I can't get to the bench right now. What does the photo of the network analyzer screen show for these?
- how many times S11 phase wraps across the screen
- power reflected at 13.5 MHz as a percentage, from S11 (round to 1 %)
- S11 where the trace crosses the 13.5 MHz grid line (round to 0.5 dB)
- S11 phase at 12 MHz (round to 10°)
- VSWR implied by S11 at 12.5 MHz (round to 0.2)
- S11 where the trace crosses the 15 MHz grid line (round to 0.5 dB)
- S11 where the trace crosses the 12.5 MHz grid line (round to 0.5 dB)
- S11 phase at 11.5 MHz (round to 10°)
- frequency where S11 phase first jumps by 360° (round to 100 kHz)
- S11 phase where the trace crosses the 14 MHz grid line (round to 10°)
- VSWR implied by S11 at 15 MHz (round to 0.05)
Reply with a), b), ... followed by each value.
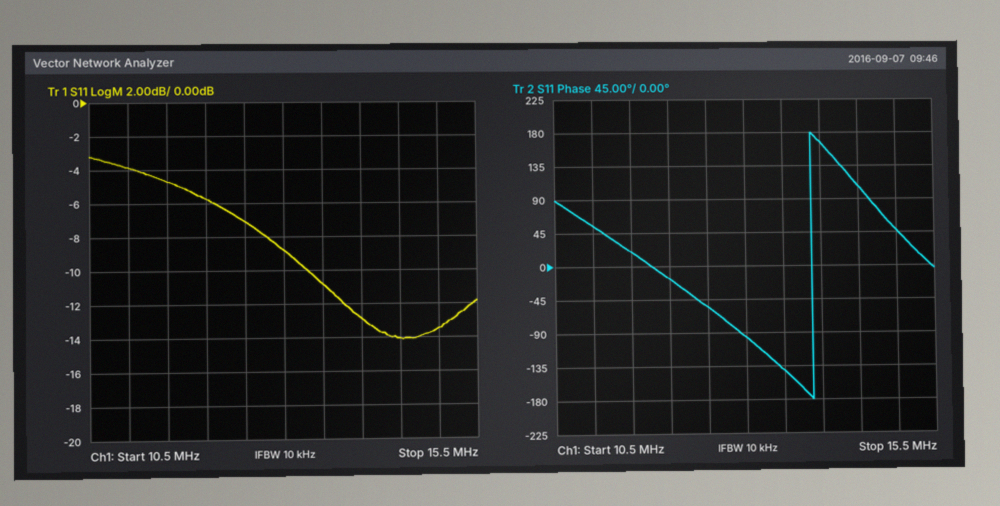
a) 1
b) 8 %
c) -11.0 dB
d) -20°
e) 2.6
f) -13.5 dB
g) -7.0 dB
h) 20°
i) 13.9 MHz
j) 170°
k) 1.55
